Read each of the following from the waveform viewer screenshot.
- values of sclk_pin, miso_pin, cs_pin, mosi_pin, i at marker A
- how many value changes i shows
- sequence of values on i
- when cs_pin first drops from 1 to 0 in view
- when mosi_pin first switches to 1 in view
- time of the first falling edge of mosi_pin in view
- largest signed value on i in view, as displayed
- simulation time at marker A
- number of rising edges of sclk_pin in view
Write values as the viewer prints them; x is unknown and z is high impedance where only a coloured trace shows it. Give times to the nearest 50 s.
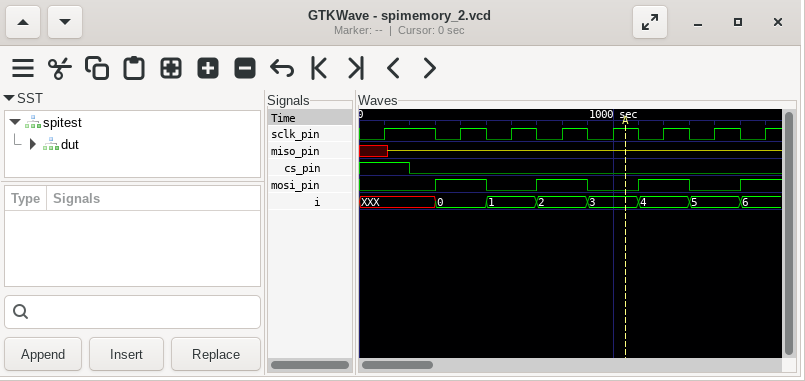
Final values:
sclk_pin=1, miso_pin=z, cs_pin=0, mosi_pin=0, i=3
7
XXX, 0, 1, 2, 3, 4, 5, 6
200 s
300 s
500 s
6
1050 s
8
